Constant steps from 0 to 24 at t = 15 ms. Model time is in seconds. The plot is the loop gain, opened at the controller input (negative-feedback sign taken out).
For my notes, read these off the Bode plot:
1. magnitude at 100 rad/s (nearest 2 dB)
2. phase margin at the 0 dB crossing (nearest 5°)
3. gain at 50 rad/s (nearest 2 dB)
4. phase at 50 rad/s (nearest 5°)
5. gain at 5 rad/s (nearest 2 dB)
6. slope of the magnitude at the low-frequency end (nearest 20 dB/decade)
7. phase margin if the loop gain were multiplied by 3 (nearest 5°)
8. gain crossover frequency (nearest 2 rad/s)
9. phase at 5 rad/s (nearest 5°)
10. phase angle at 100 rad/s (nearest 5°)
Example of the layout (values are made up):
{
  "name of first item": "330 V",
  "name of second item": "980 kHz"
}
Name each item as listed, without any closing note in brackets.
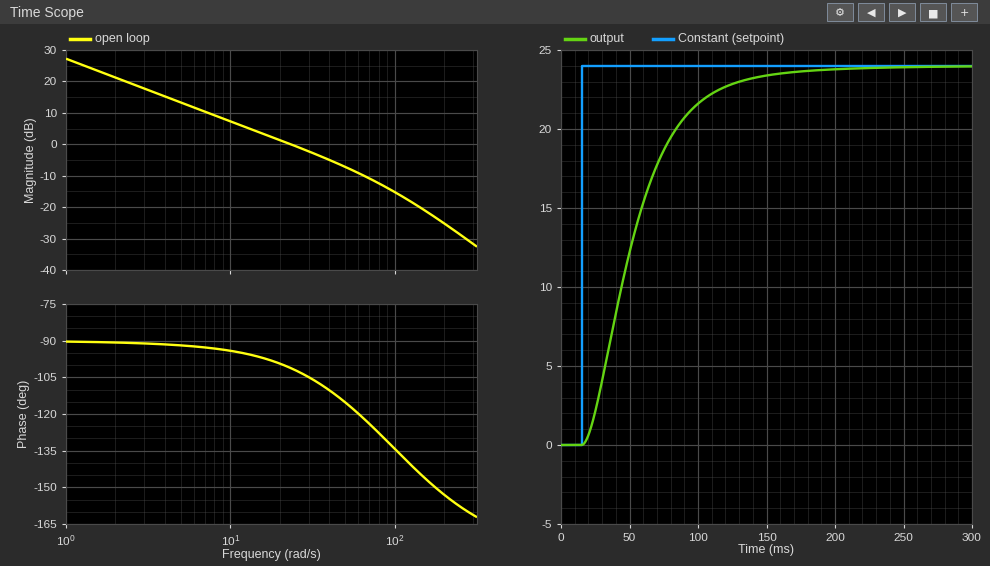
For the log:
{
  "magnitude at 100 rad/s": "-16 dB",
  "phase margin at the 0 dB crossing": "80°",
  "gain at 50 rad/s": "-8 dB",
  "phase at 50 rad/s": "-115°",
  "gain at 5 rad/s": "14 dB",
  "slope of the magnitude at the low-frequency end": "-20 dB/decade",
  "phase margin if the loop gain were multiplied by 3": "60°",
  "gain crossover frequency": "24 rad/s",
  "phase at 5 rad/s": "-90°",
  "phase angle at 100 rad/s": "-135°"
}
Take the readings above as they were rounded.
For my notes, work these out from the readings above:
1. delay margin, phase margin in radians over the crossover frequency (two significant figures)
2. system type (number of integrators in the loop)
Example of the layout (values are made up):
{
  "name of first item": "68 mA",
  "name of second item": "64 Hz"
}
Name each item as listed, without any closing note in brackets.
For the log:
{
  "delay margin, phase margin in radians over the crossover frequency": "0.058 s",
  "system type": "1"
}
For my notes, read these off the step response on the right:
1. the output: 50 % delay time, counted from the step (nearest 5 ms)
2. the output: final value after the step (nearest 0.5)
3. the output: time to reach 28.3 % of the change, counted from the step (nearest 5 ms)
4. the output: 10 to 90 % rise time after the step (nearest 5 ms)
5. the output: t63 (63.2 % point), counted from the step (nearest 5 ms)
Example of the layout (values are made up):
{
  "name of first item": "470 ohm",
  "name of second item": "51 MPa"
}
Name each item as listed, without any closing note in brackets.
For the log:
{
  "the output: 50 % delay time, counted from the step": "35 ms",
  "the output: final value after the step": "24.0",
  "the output: time to reach 28.3 % of the change, counted from the step": "20 ms",
  "the output: 10 to 90 % rise time after the step": "75 ms",
  "the output: t63 (63.2 % point), counted from the step": "45 ms"
}
